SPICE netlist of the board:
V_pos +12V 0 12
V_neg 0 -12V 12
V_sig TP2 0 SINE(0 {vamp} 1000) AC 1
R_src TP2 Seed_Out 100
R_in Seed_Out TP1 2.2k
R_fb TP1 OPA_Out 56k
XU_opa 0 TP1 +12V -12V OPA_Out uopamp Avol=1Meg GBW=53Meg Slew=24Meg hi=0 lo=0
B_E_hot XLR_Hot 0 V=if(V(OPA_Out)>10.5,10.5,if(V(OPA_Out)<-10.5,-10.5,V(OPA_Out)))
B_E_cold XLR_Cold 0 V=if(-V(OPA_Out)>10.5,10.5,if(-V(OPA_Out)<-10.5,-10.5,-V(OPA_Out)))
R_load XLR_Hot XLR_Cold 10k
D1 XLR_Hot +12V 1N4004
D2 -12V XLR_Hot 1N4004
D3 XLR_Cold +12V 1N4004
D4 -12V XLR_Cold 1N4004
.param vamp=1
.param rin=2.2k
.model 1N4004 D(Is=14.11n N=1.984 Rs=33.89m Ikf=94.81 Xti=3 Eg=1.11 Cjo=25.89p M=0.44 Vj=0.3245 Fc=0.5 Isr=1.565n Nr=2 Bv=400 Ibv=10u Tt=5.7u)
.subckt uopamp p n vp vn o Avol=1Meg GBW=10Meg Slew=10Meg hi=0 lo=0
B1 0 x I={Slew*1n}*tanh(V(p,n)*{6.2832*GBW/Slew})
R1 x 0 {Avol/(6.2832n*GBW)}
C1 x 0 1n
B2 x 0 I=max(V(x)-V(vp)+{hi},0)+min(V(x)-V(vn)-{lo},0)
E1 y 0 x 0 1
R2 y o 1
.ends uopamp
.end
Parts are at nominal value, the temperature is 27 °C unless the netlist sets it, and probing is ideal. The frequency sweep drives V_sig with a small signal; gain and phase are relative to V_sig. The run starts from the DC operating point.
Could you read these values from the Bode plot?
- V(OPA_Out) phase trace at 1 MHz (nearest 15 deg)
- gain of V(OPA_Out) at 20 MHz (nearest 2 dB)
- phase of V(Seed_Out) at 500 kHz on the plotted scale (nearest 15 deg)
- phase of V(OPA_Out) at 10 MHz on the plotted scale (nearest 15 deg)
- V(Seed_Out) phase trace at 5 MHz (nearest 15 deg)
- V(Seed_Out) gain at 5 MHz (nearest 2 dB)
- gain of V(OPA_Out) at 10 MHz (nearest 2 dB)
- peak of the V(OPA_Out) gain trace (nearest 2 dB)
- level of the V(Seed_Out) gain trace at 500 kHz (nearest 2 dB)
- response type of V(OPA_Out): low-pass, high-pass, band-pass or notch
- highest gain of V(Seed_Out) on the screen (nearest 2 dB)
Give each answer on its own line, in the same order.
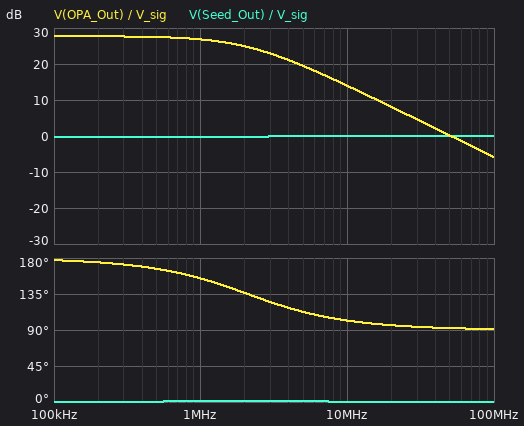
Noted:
150 deg
8 dB
0 deg
105 deg
0 deg
0 dB
14 dB
28 dB
0 dB
low-pass
0 dB
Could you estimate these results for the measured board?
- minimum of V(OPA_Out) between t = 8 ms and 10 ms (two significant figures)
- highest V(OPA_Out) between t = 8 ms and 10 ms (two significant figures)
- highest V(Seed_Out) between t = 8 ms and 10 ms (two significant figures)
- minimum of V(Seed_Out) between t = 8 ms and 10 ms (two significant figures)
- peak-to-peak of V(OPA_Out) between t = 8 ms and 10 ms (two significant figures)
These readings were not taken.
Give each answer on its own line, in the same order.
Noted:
-12 V
12 V
980 mV
-980 mV
24 V
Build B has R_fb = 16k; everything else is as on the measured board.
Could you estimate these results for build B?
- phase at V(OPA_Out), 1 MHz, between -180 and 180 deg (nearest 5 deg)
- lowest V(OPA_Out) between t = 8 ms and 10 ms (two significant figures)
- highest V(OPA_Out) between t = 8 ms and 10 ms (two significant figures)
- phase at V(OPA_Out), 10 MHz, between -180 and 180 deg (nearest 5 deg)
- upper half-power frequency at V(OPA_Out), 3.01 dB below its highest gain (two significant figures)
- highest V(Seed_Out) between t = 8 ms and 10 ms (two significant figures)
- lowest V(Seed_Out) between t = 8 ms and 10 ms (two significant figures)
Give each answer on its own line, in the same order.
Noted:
170 deg
-7.0 V
7.0 V
125 deg
6.7 MHz
960 mV
-960 mV
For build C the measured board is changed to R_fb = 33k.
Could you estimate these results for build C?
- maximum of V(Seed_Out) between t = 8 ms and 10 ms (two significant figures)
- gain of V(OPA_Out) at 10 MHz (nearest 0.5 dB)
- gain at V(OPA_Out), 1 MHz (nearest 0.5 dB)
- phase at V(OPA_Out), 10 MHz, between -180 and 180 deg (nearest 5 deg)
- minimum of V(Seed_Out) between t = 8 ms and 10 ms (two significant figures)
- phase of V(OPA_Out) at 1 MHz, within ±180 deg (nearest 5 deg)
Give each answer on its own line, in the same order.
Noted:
960 mV
13.5 dB
23.0 dB
110 deg
-960 mV
165 deg
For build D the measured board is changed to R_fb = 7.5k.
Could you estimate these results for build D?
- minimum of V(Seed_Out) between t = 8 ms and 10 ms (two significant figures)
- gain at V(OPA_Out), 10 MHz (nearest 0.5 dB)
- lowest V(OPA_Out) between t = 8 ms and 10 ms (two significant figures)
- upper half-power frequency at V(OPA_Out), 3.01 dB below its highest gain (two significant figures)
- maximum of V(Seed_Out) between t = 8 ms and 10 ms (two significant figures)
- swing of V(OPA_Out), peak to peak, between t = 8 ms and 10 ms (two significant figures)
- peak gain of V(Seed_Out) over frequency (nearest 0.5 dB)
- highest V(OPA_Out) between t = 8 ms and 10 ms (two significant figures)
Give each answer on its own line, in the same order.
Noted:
-960 mV
8.0 dB
-3.3 V
12 MHz
960 mV
6.5 V
0 dB
3.3 V
